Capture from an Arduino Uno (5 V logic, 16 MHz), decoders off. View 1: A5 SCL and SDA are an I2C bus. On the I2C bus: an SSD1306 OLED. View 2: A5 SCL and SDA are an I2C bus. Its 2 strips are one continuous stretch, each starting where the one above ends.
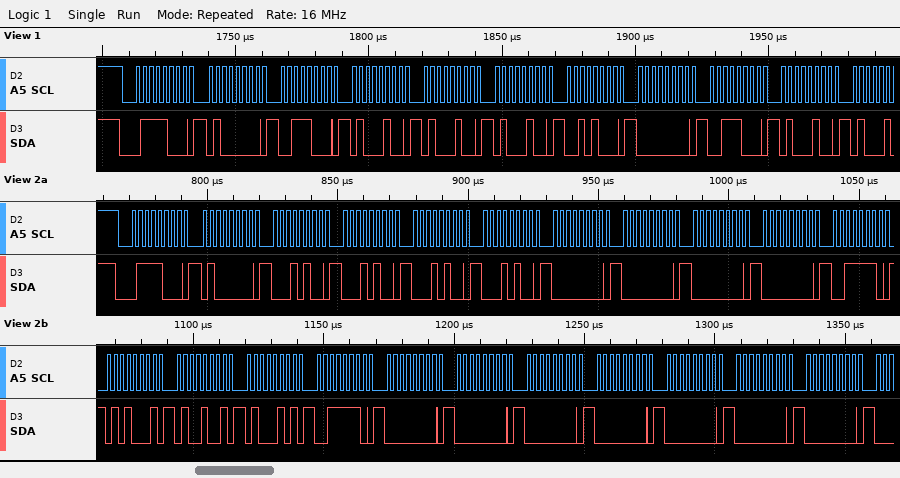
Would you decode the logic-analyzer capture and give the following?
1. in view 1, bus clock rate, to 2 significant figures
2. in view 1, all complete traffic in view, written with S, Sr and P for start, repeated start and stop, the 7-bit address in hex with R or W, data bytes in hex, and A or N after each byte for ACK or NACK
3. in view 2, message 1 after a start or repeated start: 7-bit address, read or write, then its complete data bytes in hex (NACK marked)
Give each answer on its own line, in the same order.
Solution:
400 kHz
S 3CW A 40 A 38 A 44 A 44 A 44 A 28 A 00 A 38 A 44 A
0x3C write: 40 14 14 14 14 00 00 00 00 3E 51 49 45 3E 00 00 00 00 00 00 00
